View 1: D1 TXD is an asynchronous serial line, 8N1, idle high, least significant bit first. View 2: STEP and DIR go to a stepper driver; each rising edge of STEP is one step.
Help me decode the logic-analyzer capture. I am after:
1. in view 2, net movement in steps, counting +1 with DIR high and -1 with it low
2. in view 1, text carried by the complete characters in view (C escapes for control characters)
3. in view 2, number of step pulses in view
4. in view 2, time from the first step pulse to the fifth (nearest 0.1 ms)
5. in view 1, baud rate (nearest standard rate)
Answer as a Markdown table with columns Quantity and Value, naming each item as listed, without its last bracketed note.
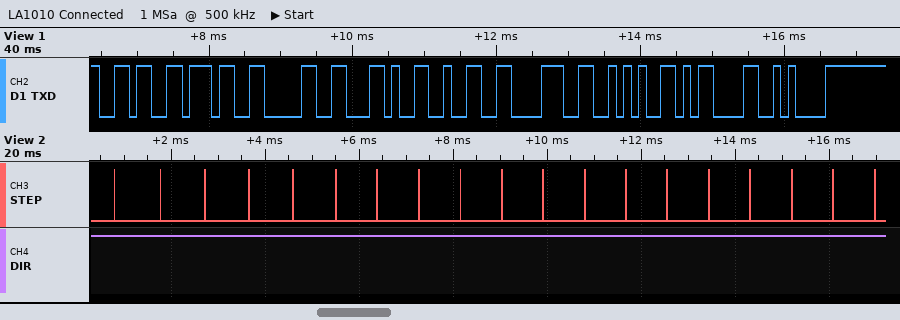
| Quantity | Value |
|---|---|
| in view 2, net movement in steps, counting +1 with DIR high and -1 with it low | +19 |
| in view 1, text carried by the complete characters in view | "670,28*\r\n" |
| in view 2, number of step pulses in view | 19 |
| in view 2, time from the first step pulse to the fifth | 3.8 ms |
| in view 1, baud rate | 9600 baud |
